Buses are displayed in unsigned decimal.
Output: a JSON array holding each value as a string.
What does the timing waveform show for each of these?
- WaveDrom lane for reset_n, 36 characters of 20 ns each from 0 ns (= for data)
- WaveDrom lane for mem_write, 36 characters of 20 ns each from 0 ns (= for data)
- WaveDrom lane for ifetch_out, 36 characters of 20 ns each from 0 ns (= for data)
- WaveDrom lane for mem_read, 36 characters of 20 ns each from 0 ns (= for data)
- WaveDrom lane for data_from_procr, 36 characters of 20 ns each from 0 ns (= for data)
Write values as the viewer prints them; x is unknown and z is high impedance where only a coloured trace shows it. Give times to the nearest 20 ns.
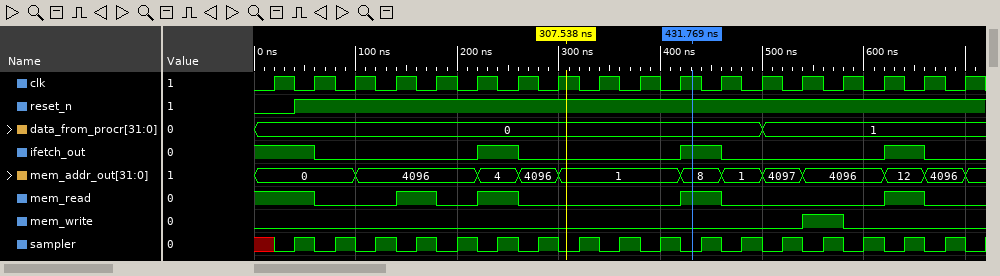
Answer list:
["{name: 'reset_n', wave: '0.1.................................'}", "{name: 'mem_write', wave: '0..........................1.0......'}", "{name: 'ifetch_out', wave: '1..0.......1.0.......1.0.......1.0..'}", "{name: 'mem_read', wave: '1..0...1.0.1.0.......1.0.......1.0..'}", "{name: 'data_from_procr', wave: '=........................=..........', data: '0 1'}"]
